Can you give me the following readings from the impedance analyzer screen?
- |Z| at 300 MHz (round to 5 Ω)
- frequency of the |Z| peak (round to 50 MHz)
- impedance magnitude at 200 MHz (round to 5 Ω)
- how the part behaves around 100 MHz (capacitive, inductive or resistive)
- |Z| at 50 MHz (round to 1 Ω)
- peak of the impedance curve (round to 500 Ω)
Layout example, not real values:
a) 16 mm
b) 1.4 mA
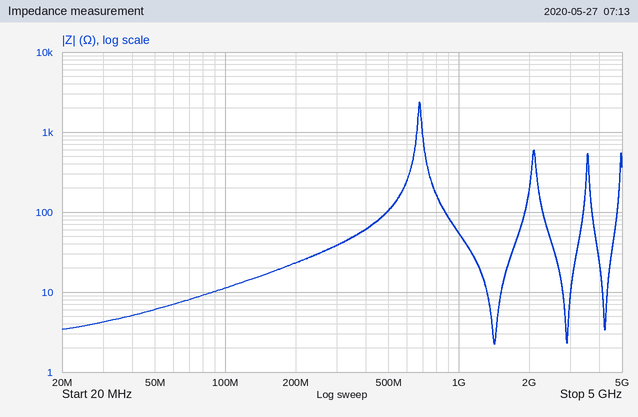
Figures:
a) 40 Ω
b) 700 MHz
c) 25 Ω
d) inductive
e) 6 Ω
f) 2.5 kΩ
